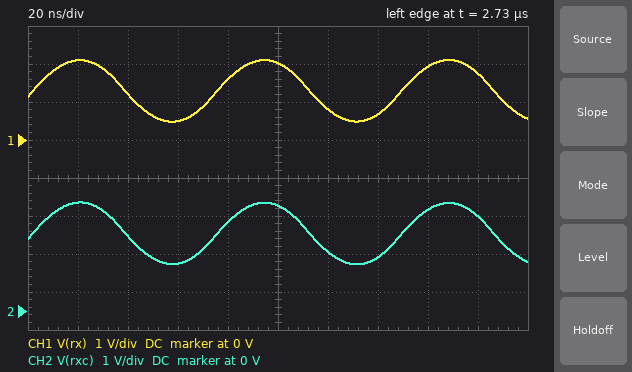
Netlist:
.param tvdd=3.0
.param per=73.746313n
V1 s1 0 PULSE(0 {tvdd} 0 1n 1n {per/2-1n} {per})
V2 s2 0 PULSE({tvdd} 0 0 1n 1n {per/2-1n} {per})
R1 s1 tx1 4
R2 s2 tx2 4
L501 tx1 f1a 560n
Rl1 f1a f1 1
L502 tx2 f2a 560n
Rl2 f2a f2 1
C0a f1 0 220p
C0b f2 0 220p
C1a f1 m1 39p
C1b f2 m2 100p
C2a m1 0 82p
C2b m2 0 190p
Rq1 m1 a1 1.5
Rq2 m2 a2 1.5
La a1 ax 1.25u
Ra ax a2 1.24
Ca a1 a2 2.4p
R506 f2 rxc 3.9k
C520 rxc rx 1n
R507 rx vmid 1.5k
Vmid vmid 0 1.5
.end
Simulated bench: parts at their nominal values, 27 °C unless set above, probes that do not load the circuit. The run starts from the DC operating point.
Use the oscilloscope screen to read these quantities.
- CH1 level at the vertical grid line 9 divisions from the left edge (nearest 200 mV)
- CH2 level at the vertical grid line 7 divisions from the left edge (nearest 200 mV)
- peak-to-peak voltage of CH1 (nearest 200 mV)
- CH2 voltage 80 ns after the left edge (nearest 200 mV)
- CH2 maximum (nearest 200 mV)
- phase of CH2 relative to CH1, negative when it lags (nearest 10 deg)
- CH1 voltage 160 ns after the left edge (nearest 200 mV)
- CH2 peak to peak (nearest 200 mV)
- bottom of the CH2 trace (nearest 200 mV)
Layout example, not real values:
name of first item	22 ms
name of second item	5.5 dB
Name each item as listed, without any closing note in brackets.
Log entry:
CH1 level at the vertical grid line 9 divisions from the left edge	1.8 V
CH2 level at the vertical grid line 7 divisions from the left edge	1.4 V
peak-to-peak voltage of CH1	1.6 V
CH2 voltage 80 ns after the left edge	2.4 V
CH2 maximum	2.8 V
phase of CH2 relative to CH1, negative when it lags	0 deg
CH1 voltage 160 ns after the left edge	2.0 V
CH2 peak to peak	1.6 V
bottom of the CH2 trace	1.2 V
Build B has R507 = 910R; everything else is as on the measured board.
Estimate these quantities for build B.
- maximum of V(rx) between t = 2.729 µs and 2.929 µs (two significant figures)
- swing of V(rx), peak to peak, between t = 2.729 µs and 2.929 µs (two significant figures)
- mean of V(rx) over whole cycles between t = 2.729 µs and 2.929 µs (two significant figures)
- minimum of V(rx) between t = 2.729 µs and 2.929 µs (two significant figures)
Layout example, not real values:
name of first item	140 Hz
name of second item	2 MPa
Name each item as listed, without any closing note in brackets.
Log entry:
maximum of V(rx) between t = 2.729 µs and 2.929 µs	1.9 V
swing of V(rx), peak to peak, between t = 2.729 µs and 2.929 µs	1.1 V
mean of V(rx) over whole cycles between t = 2.729 µs and 2.929 µs	1.4 V
minimum of V(rx) between t = 2.729 µs and 2.929 µs	810 mV
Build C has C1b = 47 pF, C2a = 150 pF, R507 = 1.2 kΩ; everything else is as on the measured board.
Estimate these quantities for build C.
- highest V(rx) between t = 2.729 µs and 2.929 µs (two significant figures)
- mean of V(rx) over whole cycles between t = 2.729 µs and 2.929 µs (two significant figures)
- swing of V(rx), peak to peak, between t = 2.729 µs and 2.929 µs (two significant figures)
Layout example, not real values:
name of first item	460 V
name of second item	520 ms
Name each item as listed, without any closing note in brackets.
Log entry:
highest V(rx) between t = 2.729 µs and 2.929 µs	1.9 V
mean of V(rx) over whole cycles between t = 2.729 µs and 2.929 µs	1.3 V
swing of V(rx), peak to peak, between t = 2.729 µs and 2.929 µs	1.1 V
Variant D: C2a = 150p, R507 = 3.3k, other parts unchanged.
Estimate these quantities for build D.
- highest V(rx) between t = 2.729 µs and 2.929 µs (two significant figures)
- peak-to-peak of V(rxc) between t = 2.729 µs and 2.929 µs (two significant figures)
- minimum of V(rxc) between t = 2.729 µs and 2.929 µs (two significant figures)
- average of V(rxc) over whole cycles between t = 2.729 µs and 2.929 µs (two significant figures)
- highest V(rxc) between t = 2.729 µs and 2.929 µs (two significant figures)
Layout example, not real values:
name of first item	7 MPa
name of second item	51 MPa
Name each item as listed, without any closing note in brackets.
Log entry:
highest V(rx) between t = 2.729 µs and 2.929 µs	2.4 V
peak-to-peak of V(rxc) between t = 2.729 µs and 2.929 µs	2.5 V
minimum of V(rxc) between t = 2.729 µs and 2.929 µs	650 mV
average of V(rxc) over whole cycles between t = 2.729 µs and 2.929 µs	1.9 V
highest V(rxc) between t = 2.729 µs and 2.929 µs	3.2 V
